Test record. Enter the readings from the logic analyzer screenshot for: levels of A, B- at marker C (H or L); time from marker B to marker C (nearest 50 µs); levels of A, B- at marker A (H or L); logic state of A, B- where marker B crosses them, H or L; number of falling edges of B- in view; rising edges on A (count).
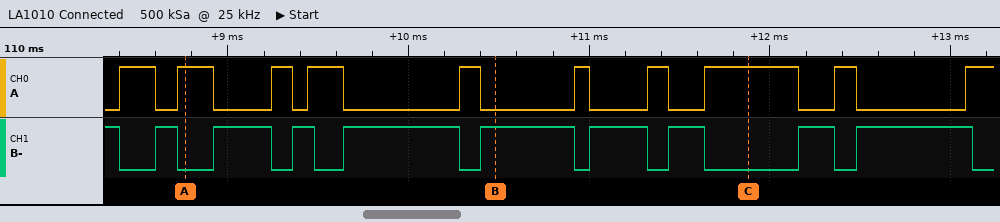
A=H, B-=L
1400 µs
A=H, B-=L
A=L, B-=H
10
10
